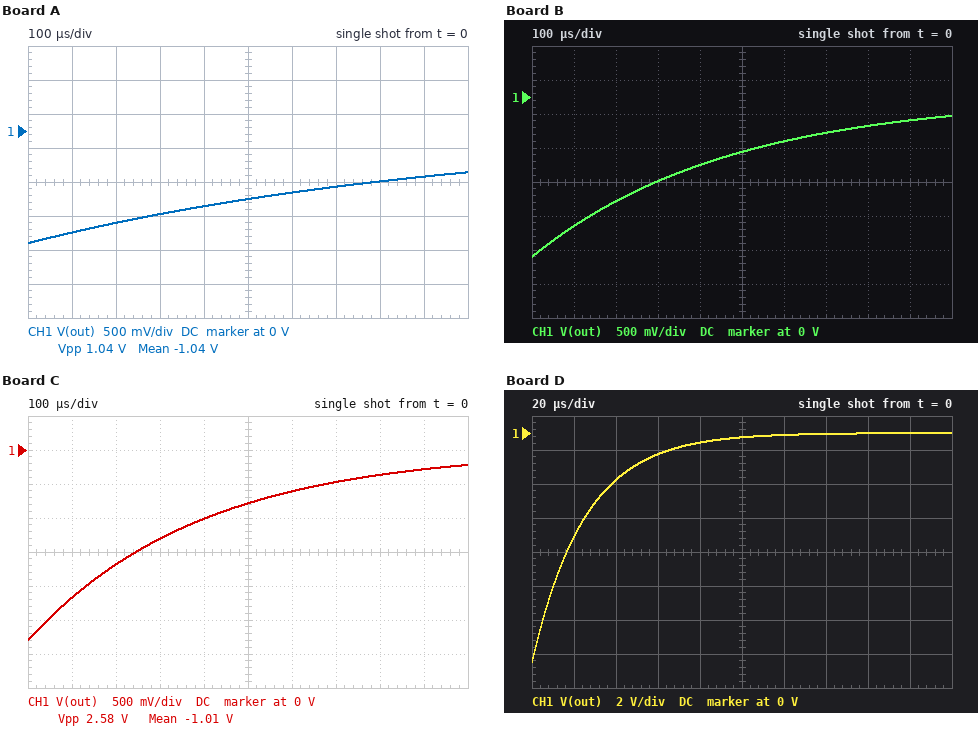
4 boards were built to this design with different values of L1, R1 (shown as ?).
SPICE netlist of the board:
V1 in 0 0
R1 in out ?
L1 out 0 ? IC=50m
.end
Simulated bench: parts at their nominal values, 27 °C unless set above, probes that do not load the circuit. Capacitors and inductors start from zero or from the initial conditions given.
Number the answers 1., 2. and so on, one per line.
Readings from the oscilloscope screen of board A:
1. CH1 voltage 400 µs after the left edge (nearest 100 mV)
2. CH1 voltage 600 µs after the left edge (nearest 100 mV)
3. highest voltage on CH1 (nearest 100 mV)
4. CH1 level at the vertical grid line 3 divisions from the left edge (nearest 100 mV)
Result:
1. -1.1 V
2. -900 mV
3. -600 mV
4. -1.2 V
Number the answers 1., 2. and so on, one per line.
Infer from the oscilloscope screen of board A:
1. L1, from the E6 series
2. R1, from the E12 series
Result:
1. 33 mH
2. 33 Ω
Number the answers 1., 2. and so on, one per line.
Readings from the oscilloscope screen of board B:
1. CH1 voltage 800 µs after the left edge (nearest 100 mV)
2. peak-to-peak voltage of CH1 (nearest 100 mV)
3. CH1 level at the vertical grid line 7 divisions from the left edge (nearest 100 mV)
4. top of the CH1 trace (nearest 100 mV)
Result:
1. -400 mV
2. 2.1 V
3. -500 mV
4. -300 mV
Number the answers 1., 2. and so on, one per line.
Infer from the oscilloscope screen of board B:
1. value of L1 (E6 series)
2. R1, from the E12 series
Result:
1. 22 mH
2. 47 Ω
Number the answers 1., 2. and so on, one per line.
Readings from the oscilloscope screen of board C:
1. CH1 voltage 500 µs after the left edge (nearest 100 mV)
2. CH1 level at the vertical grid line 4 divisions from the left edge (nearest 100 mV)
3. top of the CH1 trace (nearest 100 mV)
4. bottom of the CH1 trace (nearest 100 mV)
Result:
1. -800 mV
2. -1.0 V
3. -200 mV
4. -2.8 V
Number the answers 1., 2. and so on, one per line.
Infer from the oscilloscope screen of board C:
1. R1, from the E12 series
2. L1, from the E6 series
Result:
1. 56 Ω
2. 22 mH
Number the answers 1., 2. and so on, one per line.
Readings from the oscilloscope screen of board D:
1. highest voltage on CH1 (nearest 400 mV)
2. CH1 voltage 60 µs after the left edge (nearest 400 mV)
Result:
1. 0 V
2. -1.2 V
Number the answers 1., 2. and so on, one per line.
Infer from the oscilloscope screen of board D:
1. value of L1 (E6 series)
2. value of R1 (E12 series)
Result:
1. 6.8 mH
2. 270 Ω
